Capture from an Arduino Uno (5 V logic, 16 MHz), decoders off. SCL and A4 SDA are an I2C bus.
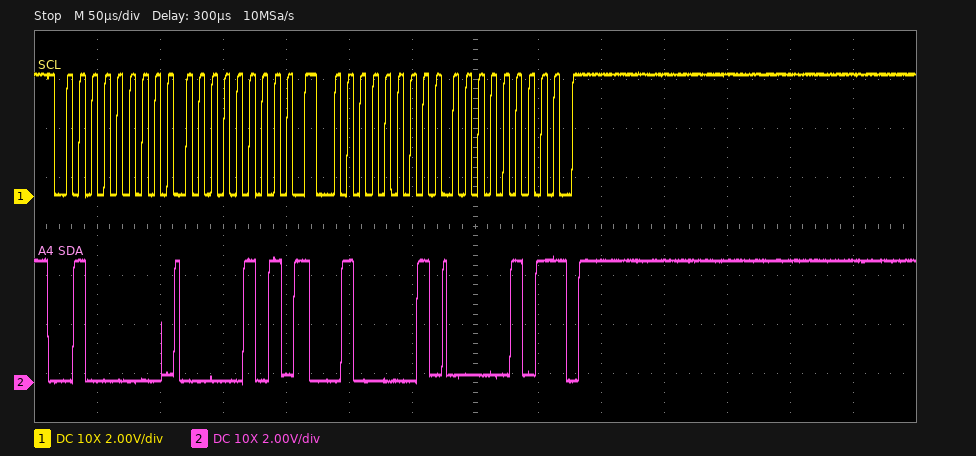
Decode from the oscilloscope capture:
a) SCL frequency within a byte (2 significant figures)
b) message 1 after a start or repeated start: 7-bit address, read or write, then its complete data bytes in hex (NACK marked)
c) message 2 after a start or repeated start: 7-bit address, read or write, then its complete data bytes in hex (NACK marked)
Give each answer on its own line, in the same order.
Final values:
100 kHz
0x20 write: 05
0x20 read: 05 NACK
